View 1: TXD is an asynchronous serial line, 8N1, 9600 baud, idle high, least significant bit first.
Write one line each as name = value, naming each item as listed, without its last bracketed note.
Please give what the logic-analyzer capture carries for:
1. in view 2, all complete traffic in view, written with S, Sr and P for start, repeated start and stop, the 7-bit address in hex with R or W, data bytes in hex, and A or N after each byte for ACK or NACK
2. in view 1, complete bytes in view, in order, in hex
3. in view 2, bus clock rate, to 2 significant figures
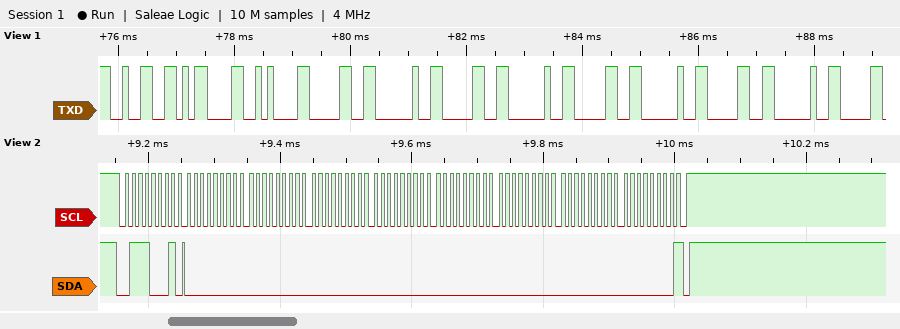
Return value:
in view 2, all complete traffic in view, written with S, Sr and P for start, repeated start and stop, the 7-bit address in hex with R or W, data bytes in hex, and A or N after each byte for ACK or NACK = S 38R A 00 A 00 A 00 A 00 A 00 A 00 A 00 A 00 N P
in view 1, complete bytes in view, in order, in hex = 32 0D 0A 30 20 30 20 30 20 30 20
in view 2, bus clock rate, to 2 significant figures = 100 kHz
